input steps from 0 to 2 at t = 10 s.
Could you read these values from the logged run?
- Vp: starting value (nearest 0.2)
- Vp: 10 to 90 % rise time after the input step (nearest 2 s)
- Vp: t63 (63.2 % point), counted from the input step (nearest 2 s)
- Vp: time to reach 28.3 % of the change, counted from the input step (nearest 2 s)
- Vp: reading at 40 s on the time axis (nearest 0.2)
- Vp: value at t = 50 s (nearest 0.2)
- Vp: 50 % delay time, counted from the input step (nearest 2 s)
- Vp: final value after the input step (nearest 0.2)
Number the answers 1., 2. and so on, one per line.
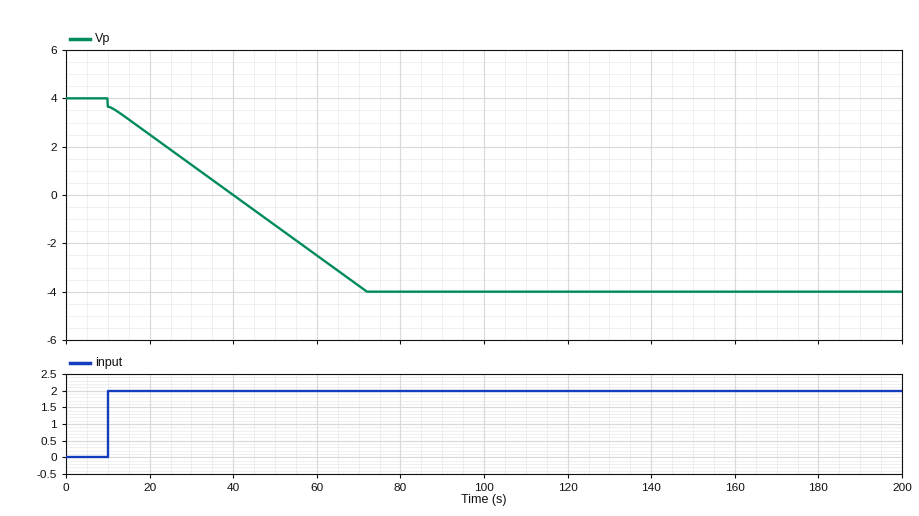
1. 4.0
2. 52 s
3. 38 s
4. 16 s
5. 0.0
6. -1.2
7. 30 s
8. -4.0
